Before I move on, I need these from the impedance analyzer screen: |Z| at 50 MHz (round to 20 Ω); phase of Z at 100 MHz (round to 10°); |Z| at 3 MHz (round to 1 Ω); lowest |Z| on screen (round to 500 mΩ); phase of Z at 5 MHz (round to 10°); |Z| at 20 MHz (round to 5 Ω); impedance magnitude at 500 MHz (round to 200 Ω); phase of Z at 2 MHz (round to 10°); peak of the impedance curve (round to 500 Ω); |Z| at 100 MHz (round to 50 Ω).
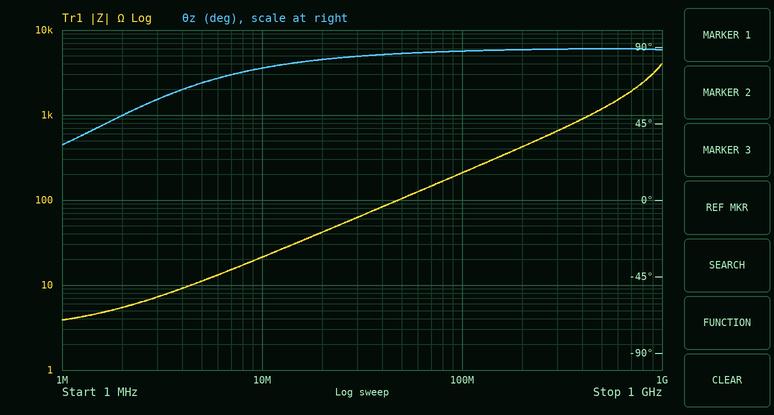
100 Ω
90°
7 Ω
4.0 Ω
70°
40 Ω
1.2 kΩ
50°
4.0 kΩ
200 Ω
